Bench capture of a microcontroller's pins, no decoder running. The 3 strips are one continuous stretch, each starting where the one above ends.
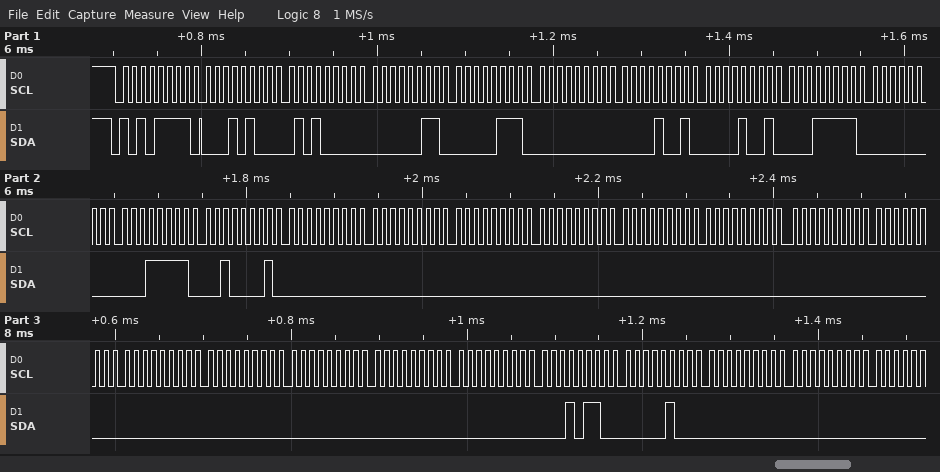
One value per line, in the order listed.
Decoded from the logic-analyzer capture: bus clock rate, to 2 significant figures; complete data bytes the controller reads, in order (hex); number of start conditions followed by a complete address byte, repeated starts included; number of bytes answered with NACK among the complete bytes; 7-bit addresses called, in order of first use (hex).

100 kHz
14 50 03 07 00 09 09 1F 00 1F 21 00 00 00 00 00 00 00 00 00 00 00 00 00 16 04 00 00
1
0
0x57
